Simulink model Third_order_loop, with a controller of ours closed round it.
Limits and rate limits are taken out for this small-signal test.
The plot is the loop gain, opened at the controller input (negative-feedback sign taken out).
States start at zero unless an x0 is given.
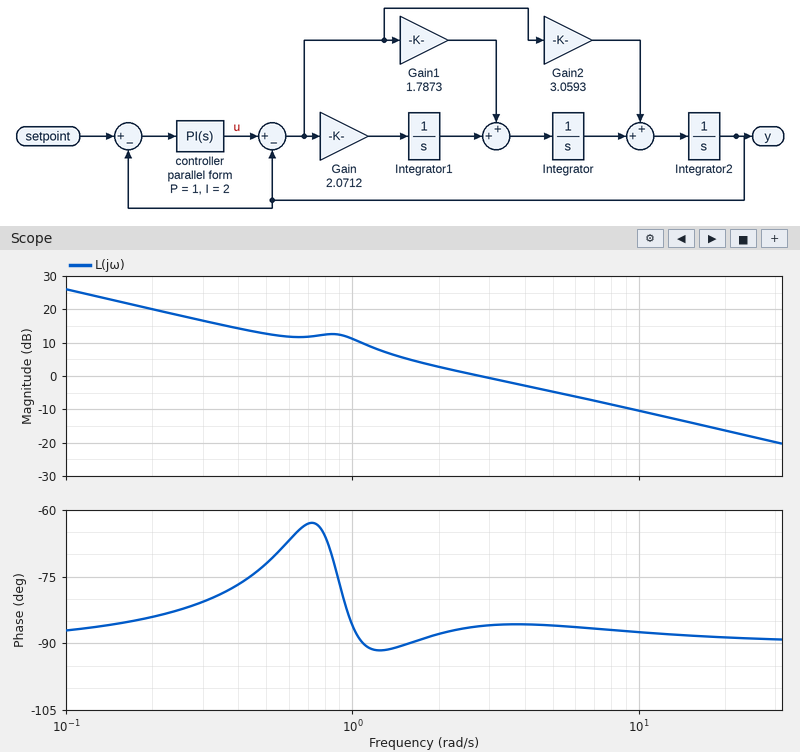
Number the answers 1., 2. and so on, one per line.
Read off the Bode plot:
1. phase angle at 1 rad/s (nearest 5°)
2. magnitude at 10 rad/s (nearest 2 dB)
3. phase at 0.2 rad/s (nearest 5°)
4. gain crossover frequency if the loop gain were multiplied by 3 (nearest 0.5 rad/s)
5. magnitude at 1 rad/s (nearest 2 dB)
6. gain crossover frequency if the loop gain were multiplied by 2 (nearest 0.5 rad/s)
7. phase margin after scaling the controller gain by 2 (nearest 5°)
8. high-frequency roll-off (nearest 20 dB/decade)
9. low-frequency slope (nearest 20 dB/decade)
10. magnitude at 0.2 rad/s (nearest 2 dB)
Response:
1. -85°
2. -10 dB
3. -85°
4. 9.0 rad/s
5. 12 dB
6. 6.0 rad/s
7. 95°
8. -20 dB/decade
9. -20 dB/decade
10. 20 dB
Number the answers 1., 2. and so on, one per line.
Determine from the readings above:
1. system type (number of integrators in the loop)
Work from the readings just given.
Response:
1. 1
